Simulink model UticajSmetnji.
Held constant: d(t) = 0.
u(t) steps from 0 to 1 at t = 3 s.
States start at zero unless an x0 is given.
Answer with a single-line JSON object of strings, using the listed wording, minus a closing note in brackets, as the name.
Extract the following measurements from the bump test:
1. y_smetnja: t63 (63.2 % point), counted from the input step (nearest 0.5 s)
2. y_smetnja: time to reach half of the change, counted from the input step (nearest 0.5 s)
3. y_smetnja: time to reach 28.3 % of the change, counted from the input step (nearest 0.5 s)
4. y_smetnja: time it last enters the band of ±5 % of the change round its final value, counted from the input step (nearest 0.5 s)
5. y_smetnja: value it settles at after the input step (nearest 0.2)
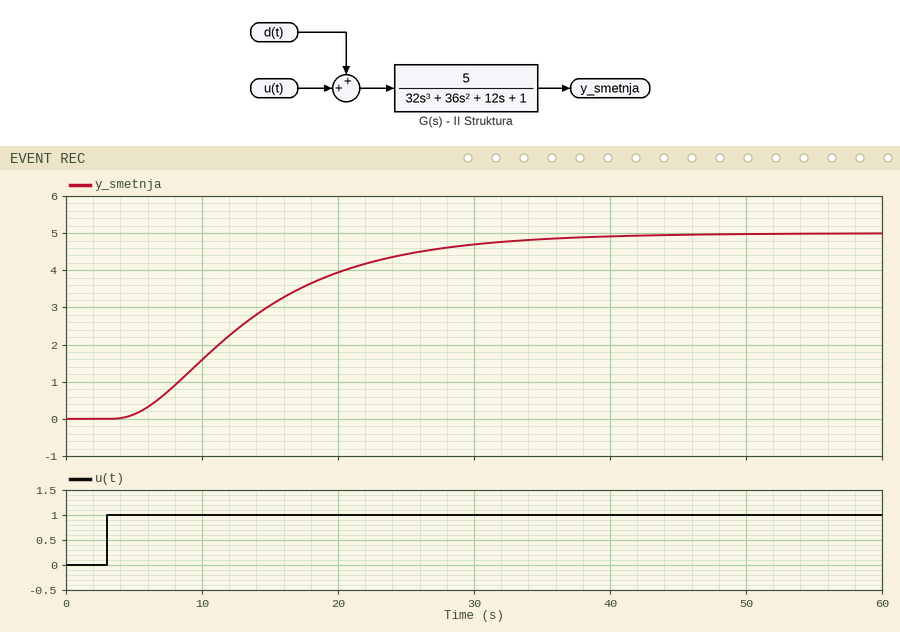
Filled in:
{"y_smetnja: t63 (63.2 % point), counted from the input step": "12.5 s", "y_smetnja: time to reach half of the change, counted from the input step": "10.0 s", "y_smetnja: time to reach 28.3 % of the change, counted from the input step": "6.5 s", "y_smetnja: time it last enters the band of ±5 % of the change round its final value, counted from the input step": "28.5 s", "y_smetnja: value it settles at after the input step": "5.0"}
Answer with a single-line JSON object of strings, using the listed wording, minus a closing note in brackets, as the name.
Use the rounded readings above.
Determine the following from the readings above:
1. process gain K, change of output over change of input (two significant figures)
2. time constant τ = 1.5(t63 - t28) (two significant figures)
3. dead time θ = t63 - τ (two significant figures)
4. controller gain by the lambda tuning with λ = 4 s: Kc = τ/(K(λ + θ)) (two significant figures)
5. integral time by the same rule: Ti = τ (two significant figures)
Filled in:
{"process gain K, change of output over change of input": "5.0", "time constant τ = 1.5(t63 - t28)": "9.0 s", "dead time θ = t63 - τ": "3.5 s", "controller gain by the lambda tuning with λ = 4 s: Kc = τ/(K(λ + θ))": "0.24", "integral time by the same rule: Ti = τ": "9.0 s"}
